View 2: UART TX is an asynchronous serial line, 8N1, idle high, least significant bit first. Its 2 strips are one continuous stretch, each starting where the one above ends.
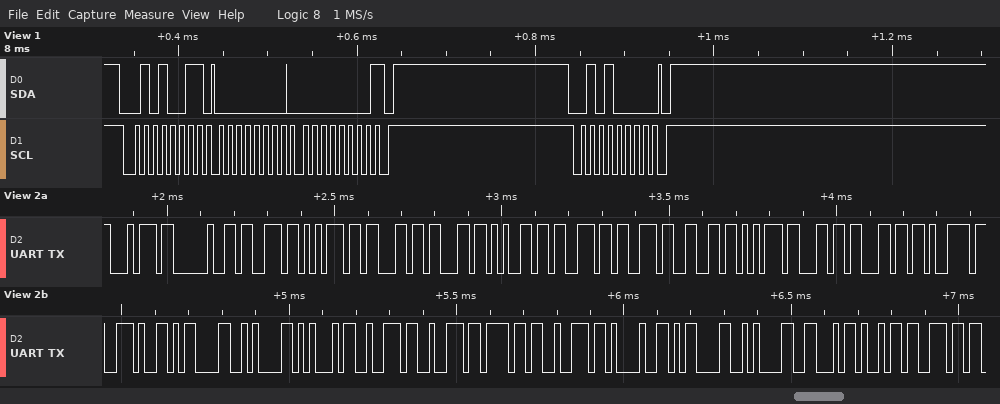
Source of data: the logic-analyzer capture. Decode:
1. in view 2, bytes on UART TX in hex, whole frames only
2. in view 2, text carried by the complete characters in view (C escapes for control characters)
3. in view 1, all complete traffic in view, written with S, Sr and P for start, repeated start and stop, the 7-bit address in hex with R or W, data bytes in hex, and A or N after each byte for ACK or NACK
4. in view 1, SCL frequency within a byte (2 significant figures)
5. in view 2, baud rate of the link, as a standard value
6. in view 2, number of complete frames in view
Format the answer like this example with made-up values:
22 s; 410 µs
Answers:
0x74 0x20 0x73 0x75 0x63 0x63 0x65 0x73 0x73 0x66 0x75 0x6C 0x6C 0x79 0x2E 0x0D 0x0A 0x45 0x72 0x72 0x6F 0x72 0x21 0x0D 0x0A 0x46 0x69 0x6E; "t successfully.\r\nError!\r\nFin"; S 29R A 00 A 00 N P S 28W A P; 100 kHz; 57600 baud; 28
